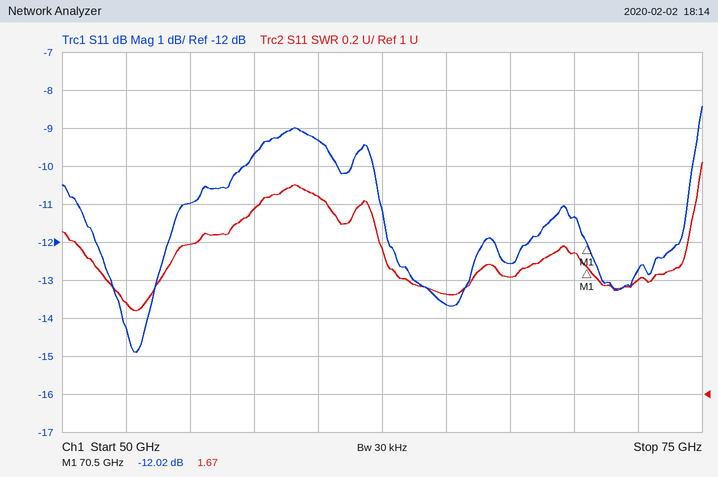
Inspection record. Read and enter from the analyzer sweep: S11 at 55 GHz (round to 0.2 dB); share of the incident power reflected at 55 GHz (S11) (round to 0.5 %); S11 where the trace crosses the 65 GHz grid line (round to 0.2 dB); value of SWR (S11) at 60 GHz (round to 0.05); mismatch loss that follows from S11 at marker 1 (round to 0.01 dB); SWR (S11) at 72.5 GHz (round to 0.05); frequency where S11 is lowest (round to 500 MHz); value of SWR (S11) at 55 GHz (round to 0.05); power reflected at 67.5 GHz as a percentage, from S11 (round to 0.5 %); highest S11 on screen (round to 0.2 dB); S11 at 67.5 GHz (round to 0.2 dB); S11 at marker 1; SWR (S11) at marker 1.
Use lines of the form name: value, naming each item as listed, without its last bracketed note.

S11 at 55 GHz: -11.0 dB
share of the incident power reflected at 55 GHz (S11): 8.0 %
S11 where the trace crosses the 65 GHz grid line: -13.6 dB
value of SWR (S11) at 60 GHz: 2.05
mismatch loss that follows from S11 at marker 1: 0.28 dB
SWR (S11) at 72.5 GHz: 1.60
frequency where S11 is lowest: 53.0 GHz
value of SWR (S11) at 55 GHz: 1.80
power reflected at 67.5 GHz as a percentage, from S11: 5.5 %
highest S11 on screen: -8.4 dB
S11 at 67.5 GHz: -12.6 dB
S11 at marker 1: -12.02 dB
SWR (S11) at marker 1: 1.67
